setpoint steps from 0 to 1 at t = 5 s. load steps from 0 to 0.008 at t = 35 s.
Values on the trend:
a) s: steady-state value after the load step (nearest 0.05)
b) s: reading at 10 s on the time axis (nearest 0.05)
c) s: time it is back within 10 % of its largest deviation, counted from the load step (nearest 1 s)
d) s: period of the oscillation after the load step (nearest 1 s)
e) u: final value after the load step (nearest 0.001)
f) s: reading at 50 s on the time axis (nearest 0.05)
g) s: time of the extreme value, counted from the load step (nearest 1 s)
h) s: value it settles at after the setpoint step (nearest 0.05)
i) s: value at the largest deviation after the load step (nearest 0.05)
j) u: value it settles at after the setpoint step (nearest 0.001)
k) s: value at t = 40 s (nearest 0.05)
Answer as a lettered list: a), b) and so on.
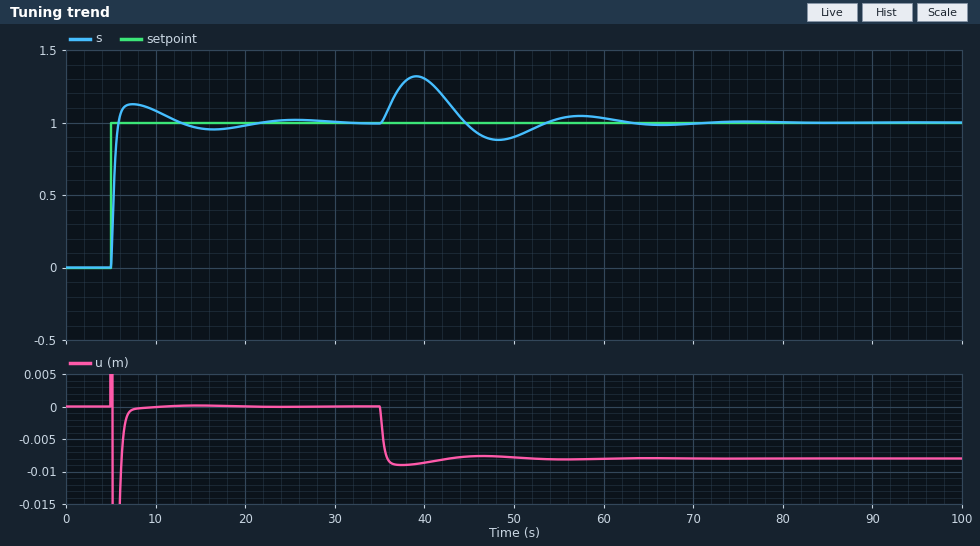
a) 1.00
b) 1.10
c) 25 s
d) 18 s
e) -0.008
f) 0.90
g) 4 s
h) 1.00
i) 1.30
j) 0.000
k) 1.30
